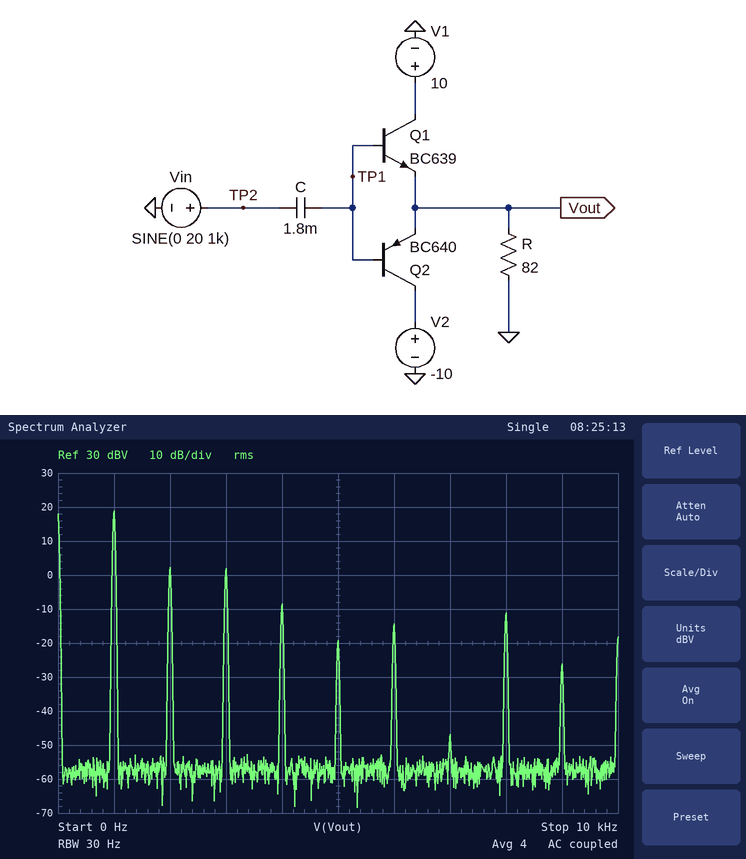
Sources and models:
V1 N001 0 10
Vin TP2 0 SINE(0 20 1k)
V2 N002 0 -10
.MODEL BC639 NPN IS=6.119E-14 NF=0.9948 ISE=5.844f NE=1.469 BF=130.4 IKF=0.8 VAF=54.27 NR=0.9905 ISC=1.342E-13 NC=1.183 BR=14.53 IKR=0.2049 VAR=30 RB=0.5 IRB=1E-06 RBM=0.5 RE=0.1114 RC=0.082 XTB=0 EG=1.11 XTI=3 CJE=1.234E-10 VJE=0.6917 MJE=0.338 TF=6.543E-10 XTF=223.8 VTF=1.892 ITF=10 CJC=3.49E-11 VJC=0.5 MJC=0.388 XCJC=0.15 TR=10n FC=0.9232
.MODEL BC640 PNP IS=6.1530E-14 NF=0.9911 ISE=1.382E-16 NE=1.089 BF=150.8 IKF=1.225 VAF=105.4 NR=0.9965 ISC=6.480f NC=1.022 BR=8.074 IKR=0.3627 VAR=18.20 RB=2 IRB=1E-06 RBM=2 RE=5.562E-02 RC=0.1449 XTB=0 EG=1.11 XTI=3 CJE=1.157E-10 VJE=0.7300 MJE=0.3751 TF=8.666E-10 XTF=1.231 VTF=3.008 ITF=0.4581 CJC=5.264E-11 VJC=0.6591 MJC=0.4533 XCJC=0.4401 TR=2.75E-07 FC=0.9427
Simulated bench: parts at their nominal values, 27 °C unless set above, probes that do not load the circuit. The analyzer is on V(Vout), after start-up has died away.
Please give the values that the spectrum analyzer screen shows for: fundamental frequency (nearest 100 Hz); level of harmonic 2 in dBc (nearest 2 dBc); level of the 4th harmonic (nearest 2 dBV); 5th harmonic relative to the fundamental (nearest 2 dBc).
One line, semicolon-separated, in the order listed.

1.0 kHz; -16 dBc; -8 dBV; -38 dBc
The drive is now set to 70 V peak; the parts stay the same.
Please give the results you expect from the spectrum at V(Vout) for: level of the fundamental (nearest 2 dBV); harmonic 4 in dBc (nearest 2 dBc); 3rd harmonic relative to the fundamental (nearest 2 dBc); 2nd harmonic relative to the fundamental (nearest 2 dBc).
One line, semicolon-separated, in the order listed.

22 dBV; -16 dBc; -20 dBc; -12 dBc
